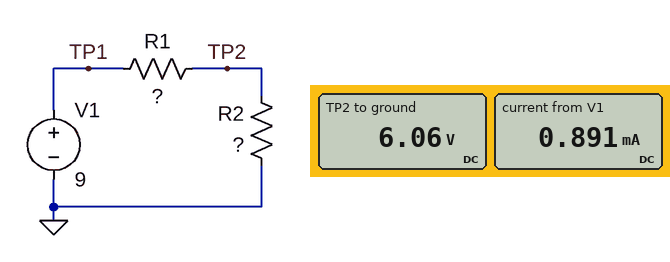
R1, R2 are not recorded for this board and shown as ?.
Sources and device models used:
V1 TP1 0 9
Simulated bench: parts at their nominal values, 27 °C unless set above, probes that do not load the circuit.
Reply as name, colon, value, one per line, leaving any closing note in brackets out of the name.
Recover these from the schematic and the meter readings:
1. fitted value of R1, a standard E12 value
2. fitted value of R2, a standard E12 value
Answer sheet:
fitted value of R1, a standard E12 value: 3.3 kΩ
fitted value of R2, a standard E12 value: 6.8 kΩ
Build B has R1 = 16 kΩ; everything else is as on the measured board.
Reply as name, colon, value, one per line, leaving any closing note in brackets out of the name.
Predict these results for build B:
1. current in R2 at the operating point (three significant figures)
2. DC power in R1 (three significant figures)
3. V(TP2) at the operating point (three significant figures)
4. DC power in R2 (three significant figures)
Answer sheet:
current in R2 at the operating point: 395 µA
DC power in R1: 2.49 mW
V(TP2) at the operating point: 2.68 V
DC power in R2: 1.06 mW
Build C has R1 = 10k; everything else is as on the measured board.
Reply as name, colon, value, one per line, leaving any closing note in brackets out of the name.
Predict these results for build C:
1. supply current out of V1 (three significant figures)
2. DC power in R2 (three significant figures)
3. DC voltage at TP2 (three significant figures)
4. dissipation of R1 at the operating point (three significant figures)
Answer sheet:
supply current out of V1: 536 µA
DC power in R2: 1.95 mW
DC voltage at TP2: 3.64 V
dissipation of R1 at the operating point: 2.87 mW
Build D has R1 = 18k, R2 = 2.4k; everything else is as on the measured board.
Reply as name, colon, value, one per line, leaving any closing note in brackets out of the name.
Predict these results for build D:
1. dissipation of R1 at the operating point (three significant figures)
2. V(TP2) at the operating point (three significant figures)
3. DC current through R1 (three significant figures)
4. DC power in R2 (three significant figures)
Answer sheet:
dissipation of R1 at the operating point: 3.50 mW
V(TP2) at the operating point: 1.06 V
DC current through R1: 441 µA
DC power in R2: 467 µW
